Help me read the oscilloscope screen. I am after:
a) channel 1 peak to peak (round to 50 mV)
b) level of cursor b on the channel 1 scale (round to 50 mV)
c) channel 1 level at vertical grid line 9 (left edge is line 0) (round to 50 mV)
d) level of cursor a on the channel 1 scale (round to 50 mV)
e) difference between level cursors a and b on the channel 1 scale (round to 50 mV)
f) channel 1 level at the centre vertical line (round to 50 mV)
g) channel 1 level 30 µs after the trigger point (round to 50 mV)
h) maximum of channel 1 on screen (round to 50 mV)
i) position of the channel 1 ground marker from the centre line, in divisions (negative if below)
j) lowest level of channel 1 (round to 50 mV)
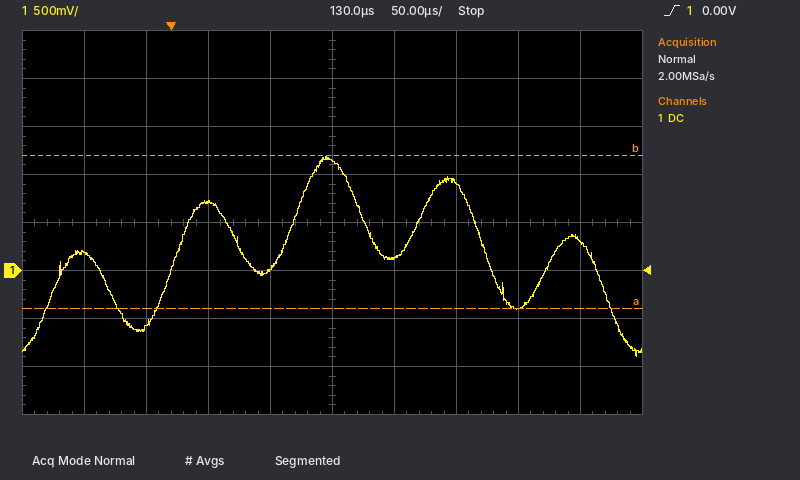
2.10 V
1.20 V
300 mV
-400 mV
1.60 V
1.15 V
700 mV
1.20 V
-1.0 div
-900 mV
